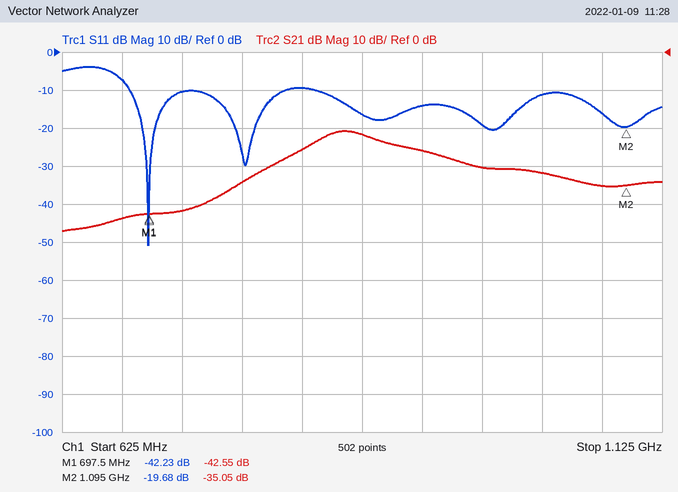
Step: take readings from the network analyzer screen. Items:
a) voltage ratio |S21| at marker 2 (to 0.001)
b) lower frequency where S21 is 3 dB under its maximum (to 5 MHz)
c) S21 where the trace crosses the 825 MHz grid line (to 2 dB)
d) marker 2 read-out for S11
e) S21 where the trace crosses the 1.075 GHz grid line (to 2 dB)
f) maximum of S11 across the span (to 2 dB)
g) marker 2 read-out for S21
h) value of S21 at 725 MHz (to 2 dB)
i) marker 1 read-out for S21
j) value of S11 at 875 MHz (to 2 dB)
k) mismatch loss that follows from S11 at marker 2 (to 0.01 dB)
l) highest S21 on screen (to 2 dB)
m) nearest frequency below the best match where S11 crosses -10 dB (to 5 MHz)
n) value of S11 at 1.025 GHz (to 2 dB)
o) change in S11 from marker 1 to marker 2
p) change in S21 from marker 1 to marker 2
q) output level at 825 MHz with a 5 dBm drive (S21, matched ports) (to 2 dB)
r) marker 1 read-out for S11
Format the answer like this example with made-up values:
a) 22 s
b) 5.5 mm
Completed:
a) 0.018
b) 835 MHz
c) -26 dB
d) -19.68 dB
e) -36 dB
f) -4 dB
g) -35.05 dB
h) -42 dB
i) -42.55 dB
j) -16 dB
k) 0.05 dB
l) -20 dB
m) 680 MHz
n) -12 dB
o) 22.55 dB
p) 7.50 dB
q) -20 dBm
r) -42.23 dB
